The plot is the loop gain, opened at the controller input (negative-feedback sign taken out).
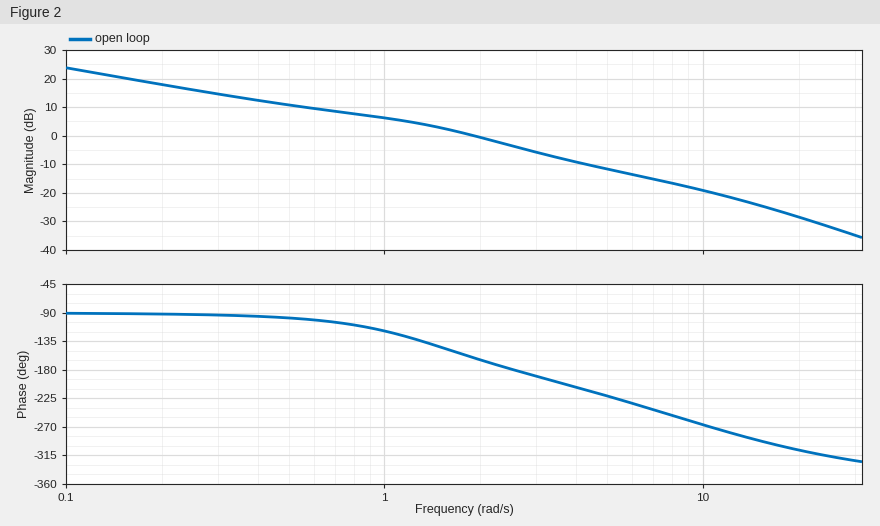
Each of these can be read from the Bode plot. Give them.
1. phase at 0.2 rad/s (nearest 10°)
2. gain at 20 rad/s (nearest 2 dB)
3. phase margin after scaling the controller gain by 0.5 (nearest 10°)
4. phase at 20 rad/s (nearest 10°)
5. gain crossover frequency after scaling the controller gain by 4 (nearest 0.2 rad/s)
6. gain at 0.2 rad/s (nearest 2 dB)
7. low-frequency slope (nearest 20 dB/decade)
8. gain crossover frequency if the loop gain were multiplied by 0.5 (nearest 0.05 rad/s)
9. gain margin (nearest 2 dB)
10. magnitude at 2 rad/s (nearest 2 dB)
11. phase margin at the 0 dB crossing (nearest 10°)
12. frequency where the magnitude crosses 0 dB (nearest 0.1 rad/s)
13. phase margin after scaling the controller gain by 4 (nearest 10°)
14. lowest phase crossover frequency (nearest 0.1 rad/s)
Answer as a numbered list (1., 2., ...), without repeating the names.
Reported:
1. -90°
2. -28 dB
3. 60°
4. -310°
5. 5.2 rad/s
6. 18 dB
7. -20 dB/decade
8. 1.05 rad/s
9. 4 dB
10. 0 dB
11. 20°
12. 1.9 rad/s
13. -40°
14. 2.5 rad/s
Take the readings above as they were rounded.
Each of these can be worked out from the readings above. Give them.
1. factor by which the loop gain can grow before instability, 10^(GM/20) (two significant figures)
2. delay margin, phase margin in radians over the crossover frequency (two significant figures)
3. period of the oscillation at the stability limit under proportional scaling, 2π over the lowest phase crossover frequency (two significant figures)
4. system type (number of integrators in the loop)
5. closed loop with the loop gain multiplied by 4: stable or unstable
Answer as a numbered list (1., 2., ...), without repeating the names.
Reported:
1. 1.6
2. 0.18 s
3. 2.5 s
4. 1
5. unstable
